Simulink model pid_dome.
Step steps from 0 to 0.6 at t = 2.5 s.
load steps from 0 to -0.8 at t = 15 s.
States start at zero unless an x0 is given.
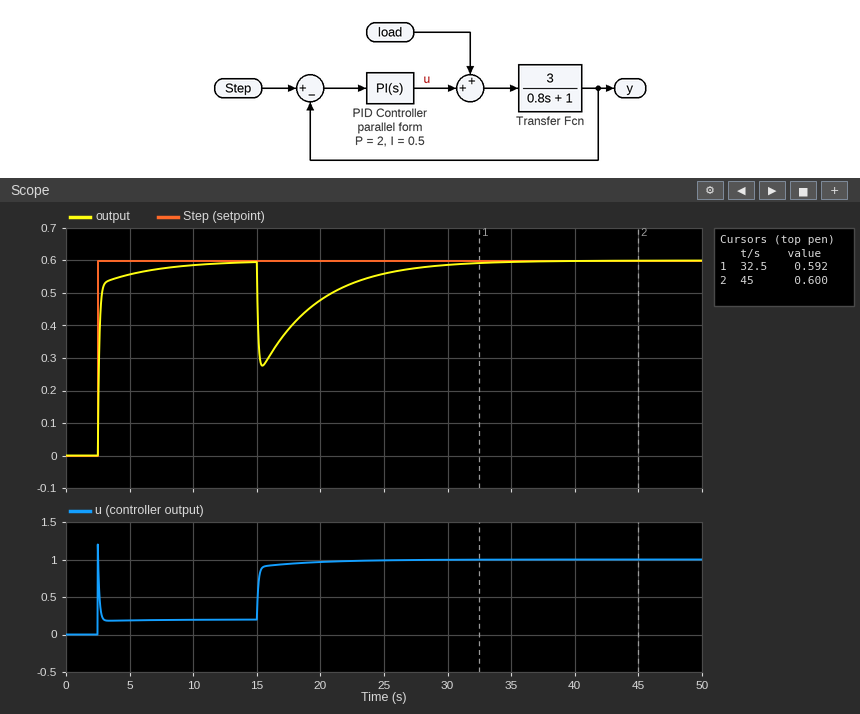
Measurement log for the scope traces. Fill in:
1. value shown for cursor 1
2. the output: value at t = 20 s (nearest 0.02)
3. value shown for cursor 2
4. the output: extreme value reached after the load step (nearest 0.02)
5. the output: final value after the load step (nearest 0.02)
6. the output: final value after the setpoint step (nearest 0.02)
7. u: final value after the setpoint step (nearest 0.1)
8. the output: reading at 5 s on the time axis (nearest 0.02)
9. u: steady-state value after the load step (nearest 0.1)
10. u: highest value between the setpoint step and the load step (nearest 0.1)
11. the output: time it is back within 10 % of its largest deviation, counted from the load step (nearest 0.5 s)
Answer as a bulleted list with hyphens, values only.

- 0.592
- 0.48
- 0.600
- 0.28
- 0.60
- 0.60
- 0.2
- 0.56
- 1.0
- 1.2
- 11.0 s
